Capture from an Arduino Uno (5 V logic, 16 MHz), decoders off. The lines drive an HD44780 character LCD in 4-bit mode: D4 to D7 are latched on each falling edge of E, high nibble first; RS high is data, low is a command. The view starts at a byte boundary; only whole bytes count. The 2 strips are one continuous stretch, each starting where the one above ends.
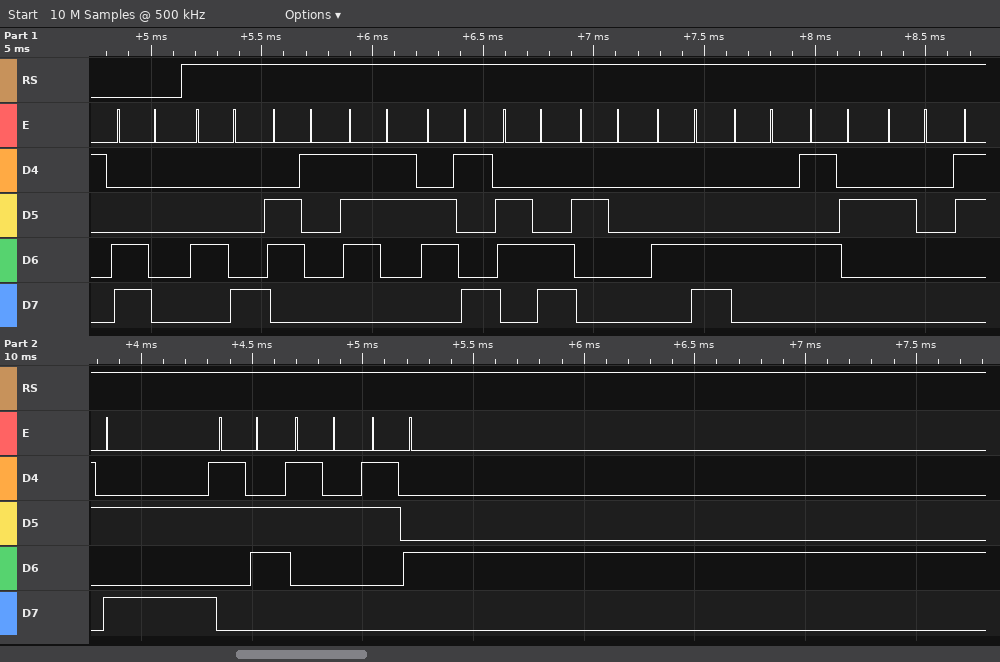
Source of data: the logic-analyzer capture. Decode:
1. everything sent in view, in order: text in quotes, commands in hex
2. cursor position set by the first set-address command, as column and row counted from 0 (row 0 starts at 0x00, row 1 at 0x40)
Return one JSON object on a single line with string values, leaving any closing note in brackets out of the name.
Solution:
{"everything sent in view, in order: text in quotes, commands in hex": "0xC0 \"Hasil LDR :624\"", "cursor position set by the first set-address command, as column and row counted from 0": "column 0, row 1"}
